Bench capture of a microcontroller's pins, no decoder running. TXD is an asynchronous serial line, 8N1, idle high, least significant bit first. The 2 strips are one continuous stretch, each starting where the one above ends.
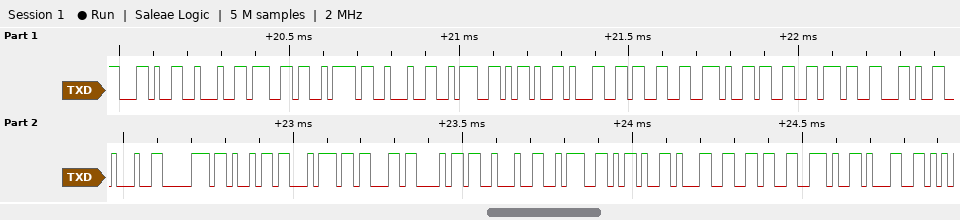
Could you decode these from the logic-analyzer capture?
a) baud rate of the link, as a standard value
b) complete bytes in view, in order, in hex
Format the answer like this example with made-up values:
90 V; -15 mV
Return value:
57600 baud; 2C 22 67 7A 22 3A 2D 31 33 2E 33 37 2C 22 70 69 74 63 68 22 3A 2D 31 36 2E 31
